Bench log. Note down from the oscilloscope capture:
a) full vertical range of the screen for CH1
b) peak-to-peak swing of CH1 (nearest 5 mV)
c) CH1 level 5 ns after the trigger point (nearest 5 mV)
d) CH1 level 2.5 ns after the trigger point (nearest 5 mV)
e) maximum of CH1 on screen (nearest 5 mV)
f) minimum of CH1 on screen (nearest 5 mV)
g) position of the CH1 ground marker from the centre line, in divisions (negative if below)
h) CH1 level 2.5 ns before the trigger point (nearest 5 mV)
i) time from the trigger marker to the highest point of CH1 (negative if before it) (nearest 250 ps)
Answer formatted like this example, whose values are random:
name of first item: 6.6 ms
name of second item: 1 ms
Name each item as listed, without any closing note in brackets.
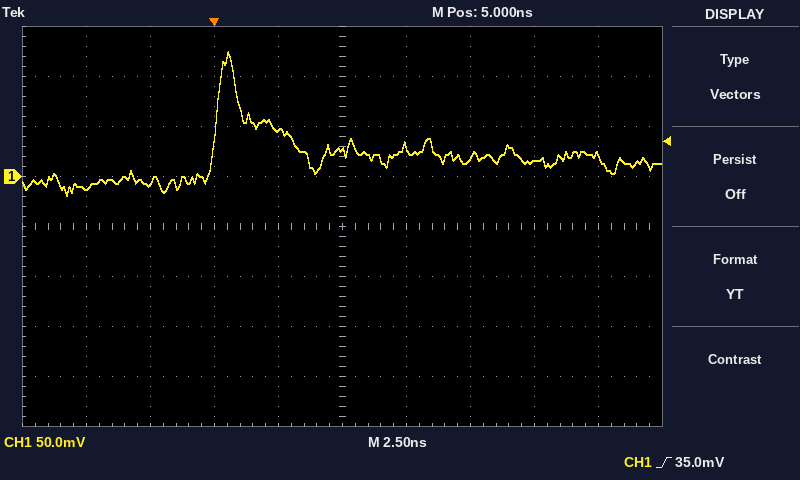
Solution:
full vertical range of the screen for CH1: 400 mV
peak-to-peak swing of CH1: 145 mV
CH1 level 5 ns after the trigger point: 25 mV
CH1 level 2.5 ns after the trigger point: 45 mV
maximum of CH1 on screen: 125 mV
minimum of CH1 on screen: -20 mV
position of the CH1 ground marker from the centre line, in divisions: +1.0 div
CH1 level 2.5 ns before the trigger point: -5 mV
time from the trigger marker to the highest point of CH1 (negative if before it): +500 ps
